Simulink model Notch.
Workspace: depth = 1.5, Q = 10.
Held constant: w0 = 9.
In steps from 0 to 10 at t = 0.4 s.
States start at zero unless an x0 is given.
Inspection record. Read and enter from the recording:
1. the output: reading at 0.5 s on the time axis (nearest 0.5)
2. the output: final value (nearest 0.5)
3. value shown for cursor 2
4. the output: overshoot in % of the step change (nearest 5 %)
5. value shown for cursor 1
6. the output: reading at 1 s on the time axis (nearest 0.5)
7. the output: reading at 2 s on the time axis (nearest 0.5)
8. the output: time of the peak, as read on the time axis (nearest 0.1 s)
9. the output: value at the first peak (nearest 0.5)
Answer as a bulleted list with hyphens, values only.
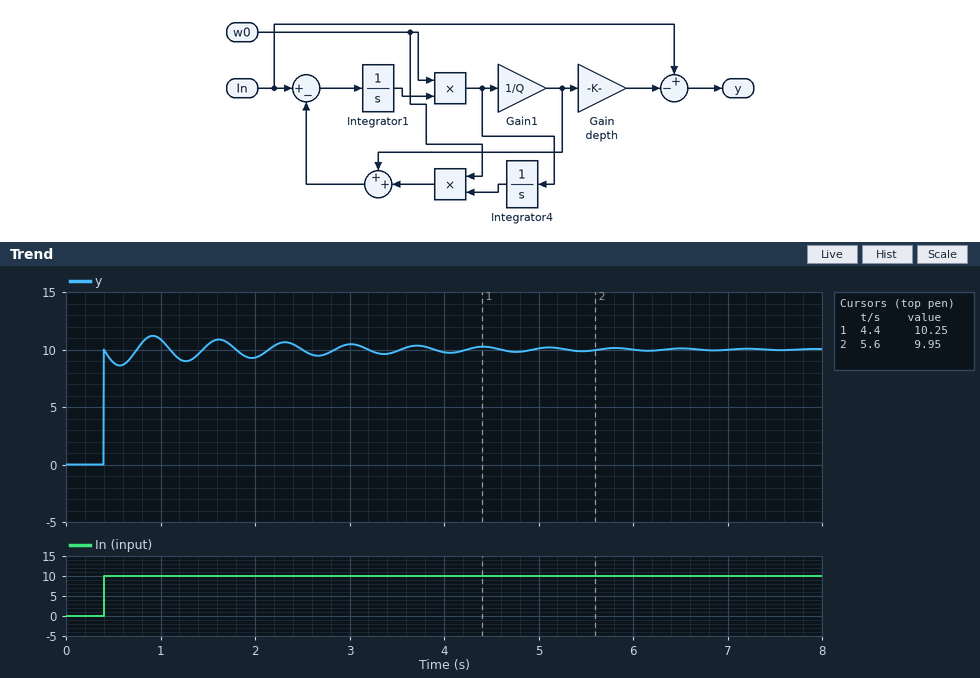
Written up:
- 9.0
- 10.0
- 9.95
- 10 %
- 10.25
- 11.0
- 9.5
- 0.9 s
- 11.0
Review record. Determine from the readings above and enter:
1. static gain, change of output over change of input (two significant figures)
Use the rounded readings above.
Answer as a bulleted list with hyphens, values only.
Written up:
- 1.0
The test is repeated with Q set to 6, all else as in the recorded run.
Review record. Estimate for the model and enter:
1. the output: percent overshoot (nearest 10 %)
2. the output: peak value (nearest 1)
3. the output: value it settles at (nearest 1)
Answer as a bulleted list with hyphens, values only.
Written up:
- 20 %
- 12
- 10
